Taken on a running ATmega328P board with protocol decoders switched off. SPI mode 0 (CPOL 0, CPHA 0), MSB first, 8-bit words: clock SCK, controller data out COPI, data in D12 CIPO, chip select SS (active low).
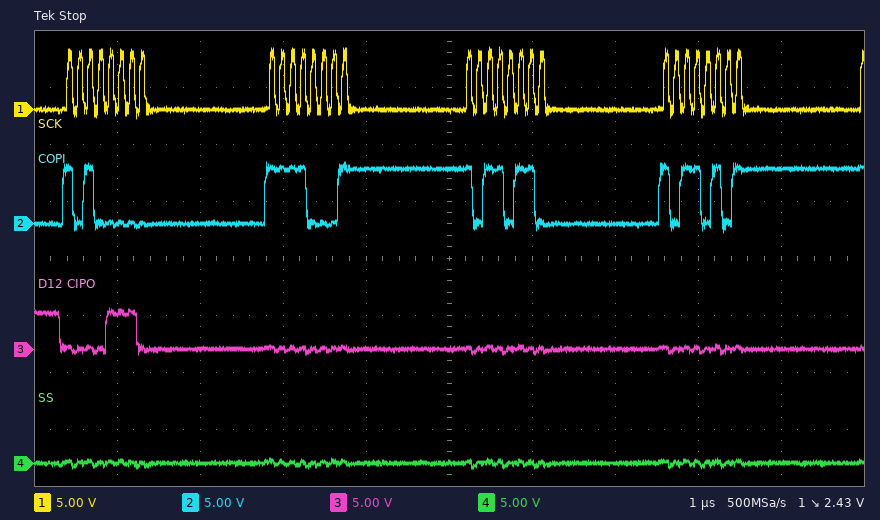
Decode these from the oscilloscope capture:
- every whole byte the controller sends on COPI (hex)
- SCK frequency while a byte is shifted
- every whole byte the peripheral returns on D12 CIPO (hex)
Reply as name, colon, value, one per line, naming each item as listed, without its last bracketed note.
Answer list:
every whole byte the controller sends on COPI: A0 F1 B6 B5
SCK frequency while a byte is shifted: 8 MHz
every whole byte the peripheral returns on D12 CIPO: 0E 00 00 00
